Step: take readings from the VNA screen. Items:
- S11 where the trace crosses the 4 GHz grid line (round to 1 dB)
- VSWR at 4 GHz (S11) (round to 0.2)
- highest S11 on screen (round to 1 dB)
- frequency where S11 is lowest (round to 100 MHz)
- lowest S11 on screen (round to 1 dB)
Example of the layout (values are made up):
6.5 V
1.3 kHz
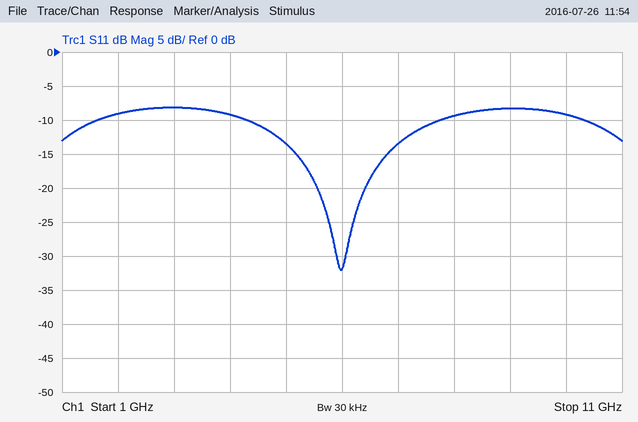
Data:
-9 dB
2.0
-8 dB
6.0 GHz
-32 dB
